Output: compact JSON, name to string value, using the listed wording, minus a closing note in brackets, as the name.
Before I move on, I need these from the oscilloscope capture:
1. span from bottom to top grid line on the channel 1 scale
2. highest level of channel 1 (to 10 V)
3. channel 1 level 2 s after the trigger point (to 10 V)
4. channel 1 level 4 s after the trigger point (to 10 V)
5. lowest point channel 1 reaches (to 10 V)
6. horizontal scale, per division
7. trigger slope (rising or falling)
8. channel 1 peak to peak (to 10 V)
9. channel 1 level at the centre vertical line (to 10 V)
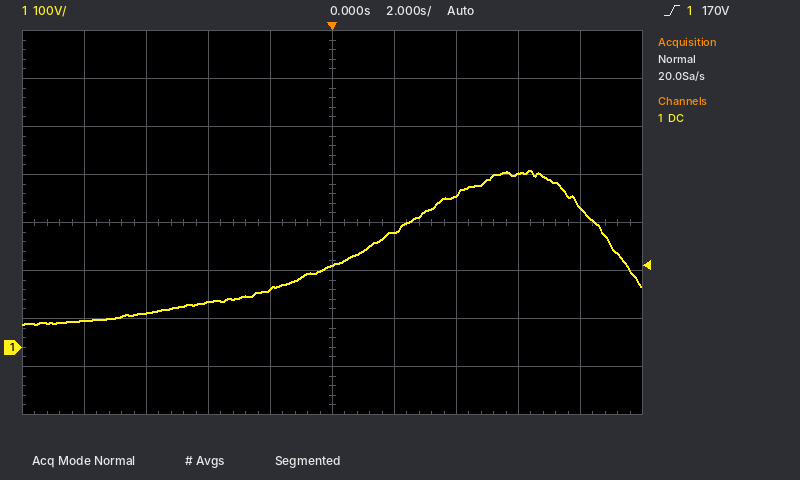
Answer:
{"span from bottom to top grid line on the channel 1 scale": "800 V", "highest level of channel 1": "370 V", "channel 1 level 2 s after the trigger point": "240 V", "channel 1 level 4 s after the trigger point": "320 V", "lowest point channel 1 reaches": "50 V", "horizontal scale, per division": "2 s", "trigger slope": "rising", "channel 1 peak to peak": "320 V", "channel 1 level at the centre vertical line": "170 V"}
